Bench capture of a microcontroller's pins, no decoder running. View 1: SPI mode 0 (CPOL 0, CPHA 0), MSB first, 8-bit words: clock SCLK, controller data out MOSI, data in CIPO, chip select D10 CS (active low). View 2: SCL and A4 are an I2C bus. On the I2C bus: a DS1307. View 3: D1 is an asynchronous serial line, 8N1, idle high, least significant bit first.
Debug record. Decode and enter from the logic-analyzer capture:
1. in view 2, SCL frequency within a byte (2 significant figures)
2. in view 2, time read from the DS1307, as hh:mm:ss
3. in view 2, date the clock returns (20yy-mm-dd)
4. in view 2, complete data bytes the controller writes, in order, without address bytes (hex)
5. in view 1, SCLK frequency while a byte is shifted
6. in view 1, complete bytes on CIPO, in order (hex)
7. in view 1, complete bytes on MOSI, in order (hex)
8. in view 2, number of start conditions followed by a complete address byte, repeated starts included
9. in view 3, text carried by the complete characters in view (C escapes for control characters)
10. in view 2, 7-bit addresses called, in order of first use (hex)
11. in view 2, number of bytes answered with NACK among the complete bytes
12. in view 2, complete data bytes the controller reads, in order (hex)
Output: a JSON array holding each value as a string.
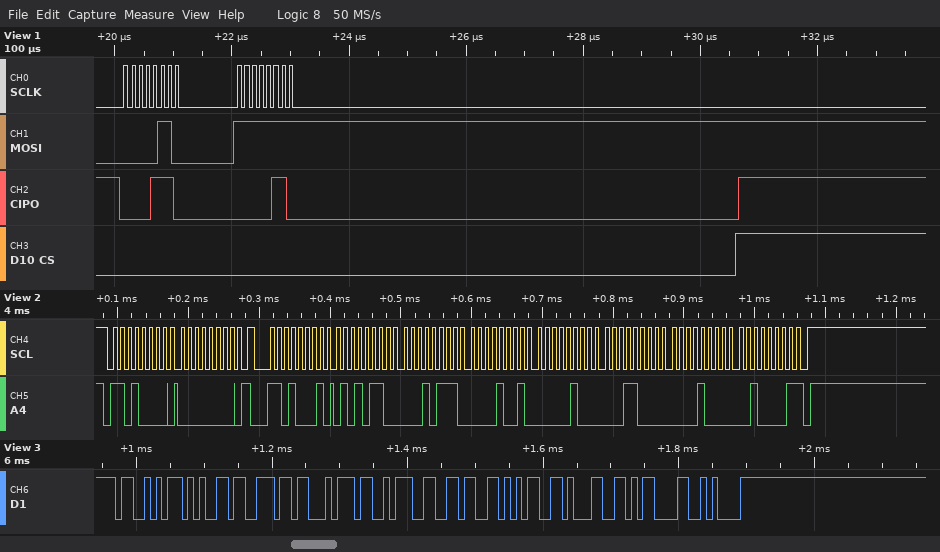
["100 kHz", "09:17:56", "2021-08-18", "00", "8 MHz", "0E 06", "06 FF", "2", "\"Sent:651\\r\\n\"", "0x68", "1", "56 17 09 04 18 08 21"]
